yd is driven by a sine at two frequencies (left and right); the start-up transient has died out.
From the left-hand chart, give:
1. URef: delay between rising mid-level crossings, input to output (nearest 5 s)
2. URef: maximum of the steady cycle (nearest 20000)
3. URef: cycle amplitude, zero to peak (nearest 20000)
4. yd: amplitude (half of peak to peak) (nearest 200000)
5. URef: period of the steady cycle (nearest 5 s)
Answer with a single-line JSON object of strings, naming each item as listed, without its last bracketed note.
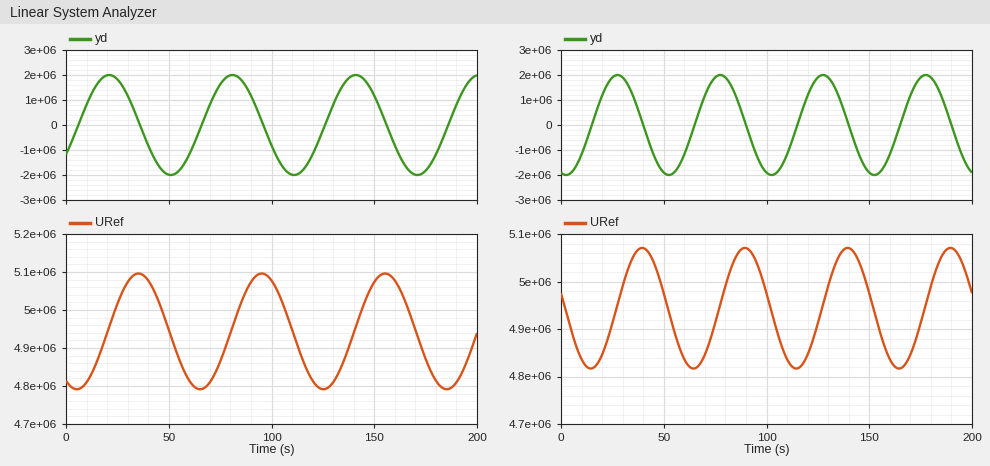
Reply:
{"URef: delay between rising mid-level crossings, input to output": "15 s", "URef: maximum of the steady cycle": "5100000", "URef: cycle amplitude, zero to peak": "160000", "yd: amplitude (half of peak to peak)": "2000000", "URef: period of the steady cycle": "60 s"}
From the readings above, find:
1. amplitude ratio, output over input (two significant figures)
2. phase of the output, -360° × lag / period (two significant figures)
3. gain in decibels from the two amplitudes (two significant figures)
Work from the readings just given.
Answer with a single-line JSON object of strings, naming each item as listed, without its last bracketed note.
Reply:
{"amplitude ratio, output over input": "0.080", "phase of the output, -360° × lag / period": "-90°", "gain in decibels from the two amplitudes": "-22 dB"}
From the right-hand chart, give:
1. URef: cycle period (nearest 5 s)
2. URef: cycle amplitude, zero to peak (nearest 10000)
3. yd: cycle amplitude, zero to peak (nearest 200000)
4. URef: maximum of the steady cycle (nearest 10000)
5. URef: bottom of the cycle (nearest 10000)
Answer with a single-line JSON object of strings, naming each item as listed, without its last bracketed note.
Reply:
{"URef: cycle period": "50 s", "URef: cycle amplitude, zero to peak": "130000", "yd: cycle amplitude, zero to peak": "2000000", "URef: maximum of the steady cycle": "5070000", "URef: bottom of the cycle": "4820000"}
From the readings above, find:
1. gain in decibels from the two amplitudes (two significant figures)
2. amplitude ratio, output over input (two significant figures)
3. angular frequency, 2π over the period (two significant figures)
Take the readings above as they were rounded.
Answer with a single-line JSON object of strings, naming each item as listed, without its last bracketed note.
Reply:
{"gain in decibels from the two amplitudes": "-24 dB", "amplitude ratio, output over input": "0.065", "angular frequency, 2π over the period": "0.13 rad/s"}
